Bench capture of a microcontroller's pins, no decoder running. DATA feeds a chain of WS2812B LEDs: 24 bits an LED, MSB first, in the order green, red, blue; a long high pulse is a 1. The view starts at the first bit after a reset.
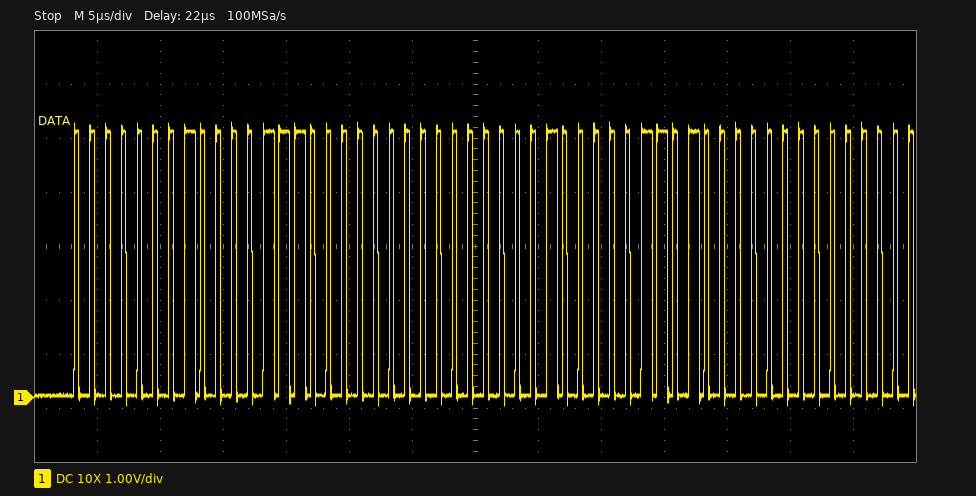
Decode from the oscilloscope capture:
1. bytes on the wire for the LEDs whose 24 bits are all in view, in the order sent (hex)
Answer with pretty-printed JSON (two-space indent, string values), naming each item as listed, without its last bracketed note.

{
  "bytes on the wire for the LEDs whose 24 bits are all in view, in the order sent": "01 0E 00 02 0D 00"
}
